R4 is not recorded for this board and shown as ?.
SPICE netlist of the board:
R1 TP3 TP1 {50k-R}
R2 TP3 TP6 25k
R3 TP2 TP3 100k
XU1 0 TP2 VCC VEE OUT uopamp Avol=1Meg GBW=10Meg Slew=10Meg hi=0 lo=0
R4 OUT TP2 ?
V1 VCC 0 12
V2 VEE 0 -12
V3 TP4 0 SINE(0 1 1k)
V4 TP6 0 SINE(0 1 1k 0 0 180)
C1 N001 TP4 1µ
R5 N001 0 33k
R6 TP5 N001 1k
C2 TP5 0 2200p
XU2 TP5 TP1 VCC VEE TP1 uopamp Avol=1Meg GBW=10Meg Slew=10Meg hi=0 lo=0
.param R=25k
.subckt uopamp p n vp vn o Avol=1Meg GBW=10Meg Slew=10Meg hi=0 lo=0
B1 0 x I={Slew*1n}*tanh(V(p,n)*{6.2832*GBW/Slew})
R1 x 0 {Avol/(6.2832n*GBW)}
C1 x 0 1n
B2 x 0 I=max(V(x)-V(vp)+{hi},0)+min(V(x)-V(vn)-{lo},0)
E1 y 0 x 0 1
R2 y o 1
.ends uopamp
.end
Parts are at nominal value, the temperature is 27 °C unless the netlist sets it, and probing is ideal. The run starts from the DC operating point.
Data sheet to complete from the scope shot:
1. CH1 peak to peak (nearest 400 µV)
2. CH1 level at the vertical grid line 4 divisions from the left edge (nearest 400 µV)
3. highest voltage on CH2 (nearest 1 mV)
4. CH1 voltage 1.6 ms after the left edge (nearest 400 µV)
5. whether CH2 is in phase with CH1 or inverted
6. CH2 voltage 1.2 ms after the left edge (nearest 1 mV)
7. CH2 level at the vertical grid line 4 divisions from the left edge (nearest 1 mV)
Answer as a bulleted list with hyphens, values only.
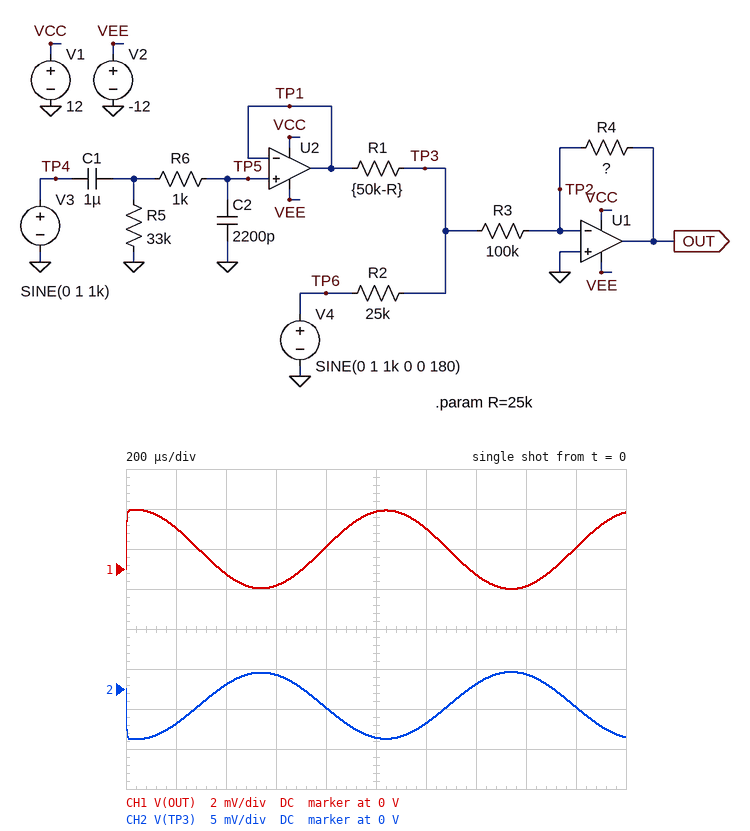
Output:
- 4.0 mV
- 1.2 mV
- 2 mV
- -800 µV
- inverted
- -4 mV
- -2 mV
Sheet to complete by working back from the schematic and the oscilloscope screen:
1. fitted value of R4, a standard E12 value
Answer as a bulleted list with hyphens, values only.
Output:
- 47 kΩ
